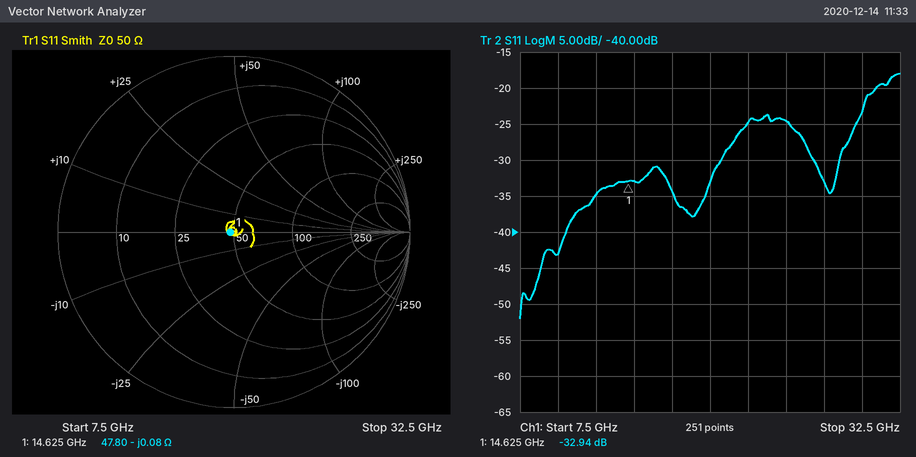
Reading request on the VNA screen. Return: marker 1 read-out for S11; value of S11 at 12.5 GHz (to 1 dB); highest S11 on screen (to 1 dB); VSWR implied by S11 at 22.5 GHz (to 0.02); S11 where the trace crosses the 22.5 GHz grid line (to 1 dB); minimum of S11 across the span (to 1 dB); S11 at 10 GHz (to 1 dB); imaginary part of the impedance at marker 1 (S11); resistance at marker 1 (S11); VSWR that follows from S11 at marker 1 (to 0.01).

-32.94 dB
-35 dB
-18 dB
1.12
-25 dB
-52 dB
-43 dB
-0.08 Ω
47.80 Ω
1.05
